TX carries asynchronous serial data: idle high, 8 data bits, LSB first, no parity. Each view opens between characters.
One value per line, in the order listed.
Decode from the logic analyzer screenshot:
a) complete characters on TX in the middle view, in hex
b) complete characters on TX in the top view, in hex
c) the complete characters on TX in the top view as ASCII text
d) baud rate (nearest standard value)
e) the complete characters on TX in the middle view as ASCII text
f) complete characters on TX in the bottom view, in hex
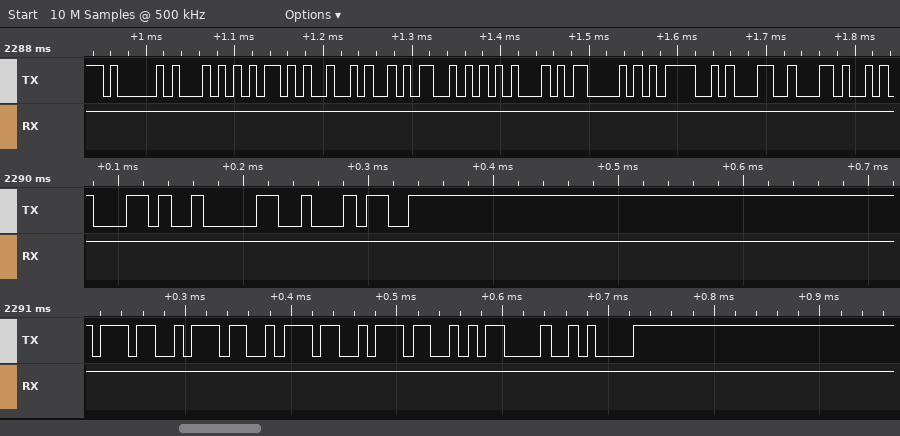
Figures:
2C, 30, 34
41, 54, 2B, 4A, 53, 45, 43, 3D, 31, 2C
"AT+JSEC=1,"
115200 baud
",04"
37, 37, 37, 37, 0D, 0A
